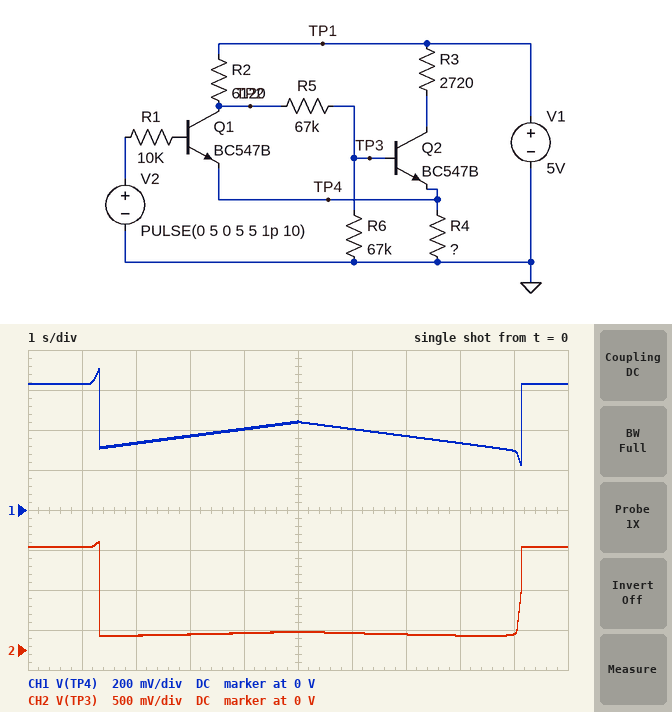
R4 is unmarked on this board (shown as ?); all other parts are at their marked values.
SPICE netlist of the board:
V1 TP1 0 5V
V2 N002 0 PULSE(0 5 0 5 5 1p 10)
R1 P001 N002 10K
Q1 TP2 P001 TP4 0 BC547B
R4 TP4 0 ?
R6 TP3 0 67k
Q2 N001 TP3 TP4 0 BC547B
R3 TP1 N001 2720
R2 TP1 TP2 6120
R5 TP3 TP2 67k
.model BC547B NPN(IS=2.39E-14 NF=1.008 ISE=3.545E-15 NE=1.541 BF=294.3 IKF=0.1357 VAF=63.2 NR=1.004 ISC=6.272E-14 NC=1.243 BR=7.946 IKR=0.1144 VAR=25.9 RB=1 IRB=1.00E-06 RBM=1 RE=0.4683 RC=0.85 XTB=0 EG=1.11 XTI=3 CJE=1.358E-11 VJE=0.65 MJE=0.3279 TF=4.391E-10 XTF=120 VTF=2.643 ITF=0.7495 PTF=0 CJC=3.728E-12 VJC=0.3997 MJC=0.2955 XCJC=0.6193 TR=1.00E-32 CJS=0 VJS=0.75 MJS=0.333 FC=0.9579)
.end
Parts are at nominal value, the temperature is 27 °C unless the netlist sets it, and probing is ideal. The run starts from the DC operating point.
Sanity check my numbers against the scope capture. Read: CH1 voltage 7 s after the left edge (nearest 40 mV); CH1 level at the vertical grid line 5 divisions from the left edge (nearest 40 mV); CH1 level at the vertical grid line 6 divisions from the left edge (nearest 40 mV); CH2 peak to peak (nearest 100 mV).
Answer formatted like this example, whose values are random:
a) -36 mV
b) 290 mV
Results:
a) 360 mV
b) 440 mV
c) 400 mV
d) 1.2 V
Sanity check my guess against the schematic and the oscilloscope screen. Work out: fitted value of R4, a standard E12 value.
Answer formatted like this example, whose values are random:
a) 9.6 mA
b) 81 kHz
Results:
a) 390 Ω
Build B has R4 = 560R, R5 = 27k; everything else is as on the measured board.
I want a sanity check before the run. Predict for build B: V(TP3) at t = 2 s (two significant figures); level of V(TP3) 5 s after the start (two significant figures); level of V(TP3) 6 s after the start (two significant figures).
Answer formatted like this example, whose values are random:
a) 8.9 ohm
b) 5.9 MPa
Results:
a) 350 mV
b) 440 mV
c) 410 mV
